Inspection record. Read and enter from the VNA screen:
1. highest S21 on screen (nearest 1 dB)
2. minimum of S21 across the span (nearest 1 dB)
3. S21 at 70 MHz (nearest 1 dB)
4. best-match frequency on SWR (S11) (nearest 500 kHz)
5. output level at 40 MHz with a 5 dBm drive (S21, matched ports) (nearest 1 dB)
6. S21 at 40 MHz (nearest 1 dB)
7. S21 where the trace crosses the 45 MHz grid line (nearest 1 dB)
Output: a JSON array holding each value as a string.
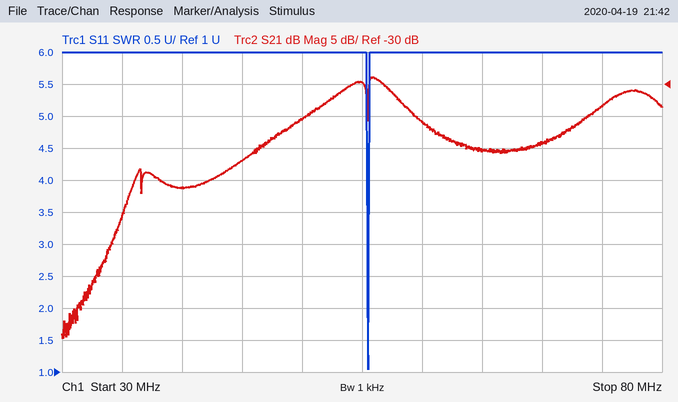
["-29 dB", "-70 dB", "-39 dB", "55.5 MHz", "-41 dBm", "-46 dB", "-42 dB"]
